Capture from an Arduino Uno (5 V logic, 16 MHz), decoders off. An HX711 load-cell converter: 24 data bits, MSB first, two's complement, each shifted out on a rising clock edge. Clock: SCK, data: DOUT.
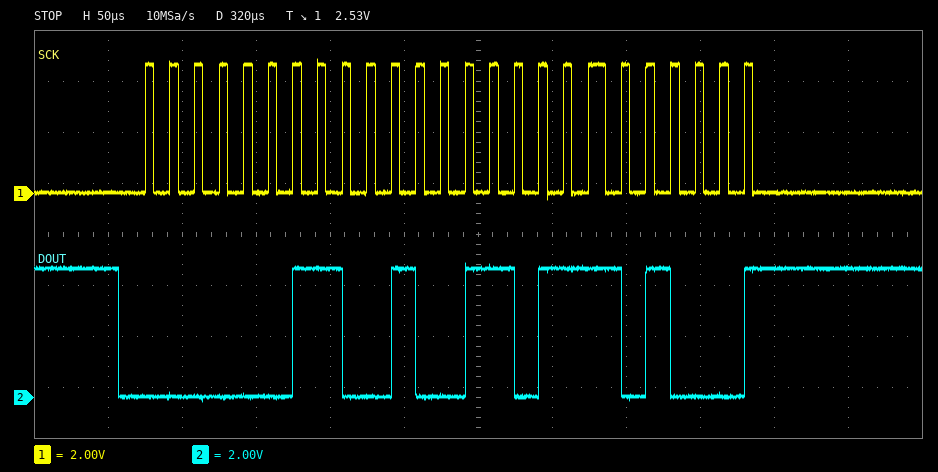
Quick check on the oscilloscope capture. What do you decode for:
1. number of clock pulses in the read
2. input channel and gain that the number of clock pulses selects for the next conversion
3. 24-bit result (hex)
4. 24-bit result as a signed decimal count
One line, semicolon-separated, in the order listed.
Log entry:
25; channel A, gain 128; 0x0326E8; 206568
